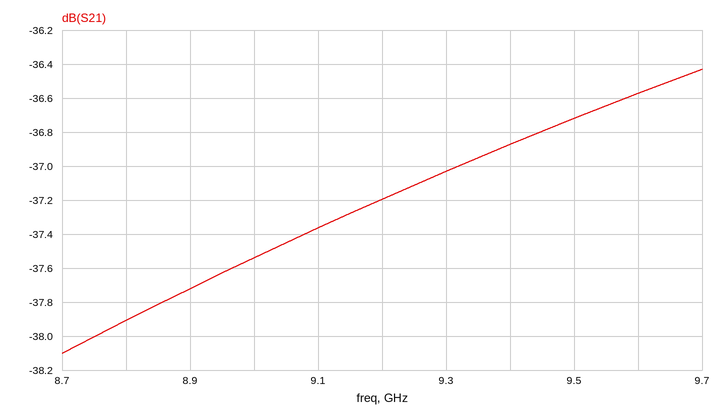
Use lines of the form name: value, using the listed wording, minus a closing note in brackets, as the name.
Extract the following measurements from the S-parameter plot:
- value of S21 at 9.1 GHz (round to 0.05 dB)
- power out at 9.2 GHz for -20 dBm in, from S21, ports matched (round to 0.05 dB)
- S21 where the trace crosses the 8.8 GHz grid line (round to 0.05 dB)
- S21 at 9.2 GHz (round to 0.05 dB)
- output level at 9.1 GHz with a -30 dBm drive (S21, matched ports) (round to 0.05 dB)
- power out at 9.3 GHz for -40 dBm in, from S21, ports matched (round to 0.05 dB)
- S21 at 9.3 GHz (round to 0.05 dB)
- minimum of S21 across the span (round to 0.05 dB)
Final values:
value of S21 at 9.1 GHz: -37.35 dB
power out at 9.2 GHz for -20 dBm in, from S21, ports matched: -57.20 dBm
S21 where the trace crosses the 8.8 GHz grid line: -37.90 dB
S21 at 9.2 GHz: -37.20 dB
output level at 9.1 GHz with a -30 dBm drive (S21, matched ports): -67.35 dBm
power out at 9.3 GHz for -40 dBm in, from S21, ports matched: -77.05 dBm
S21 at 9.3 GHz: -37.05 dB
minimum of S21 across the span: -38.10 dB
